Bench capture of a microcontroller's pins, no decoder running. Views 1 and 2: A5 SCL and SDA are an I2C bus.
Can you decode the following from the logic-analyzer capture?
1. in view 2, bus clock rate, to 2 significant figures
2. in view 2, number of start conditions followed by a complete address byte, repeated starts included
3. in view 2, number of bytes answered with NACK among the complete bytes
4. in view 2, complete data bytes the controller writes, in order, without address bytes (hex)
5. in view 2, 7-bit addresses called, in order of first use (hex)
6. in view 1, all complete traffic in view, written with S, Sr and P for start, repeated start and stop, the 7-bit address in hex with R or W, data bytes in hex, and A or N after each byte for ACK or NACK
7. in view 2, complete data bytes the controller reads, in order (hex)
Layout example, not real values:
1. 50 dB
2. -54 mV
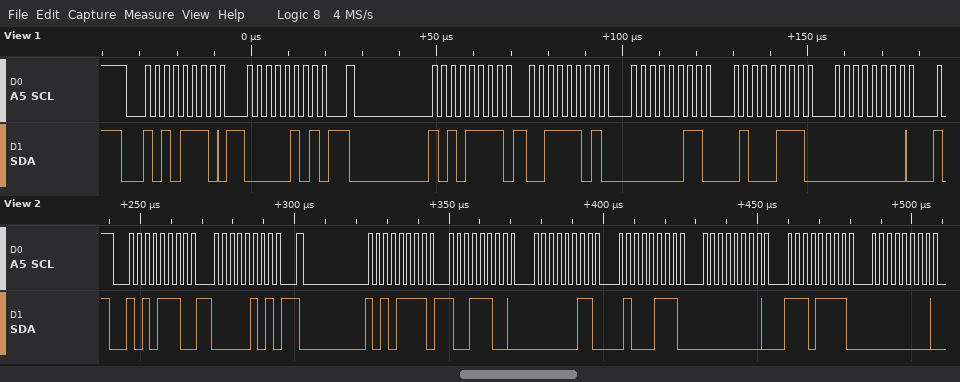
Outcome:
1. 400 kHz
2. 2
3. 0
4. 05
5. 0x57
6. S 57W A 05 A Sr 57R A 3D A 03 A 47 A 00 A
7. 9C 03 47 00 EF 00
